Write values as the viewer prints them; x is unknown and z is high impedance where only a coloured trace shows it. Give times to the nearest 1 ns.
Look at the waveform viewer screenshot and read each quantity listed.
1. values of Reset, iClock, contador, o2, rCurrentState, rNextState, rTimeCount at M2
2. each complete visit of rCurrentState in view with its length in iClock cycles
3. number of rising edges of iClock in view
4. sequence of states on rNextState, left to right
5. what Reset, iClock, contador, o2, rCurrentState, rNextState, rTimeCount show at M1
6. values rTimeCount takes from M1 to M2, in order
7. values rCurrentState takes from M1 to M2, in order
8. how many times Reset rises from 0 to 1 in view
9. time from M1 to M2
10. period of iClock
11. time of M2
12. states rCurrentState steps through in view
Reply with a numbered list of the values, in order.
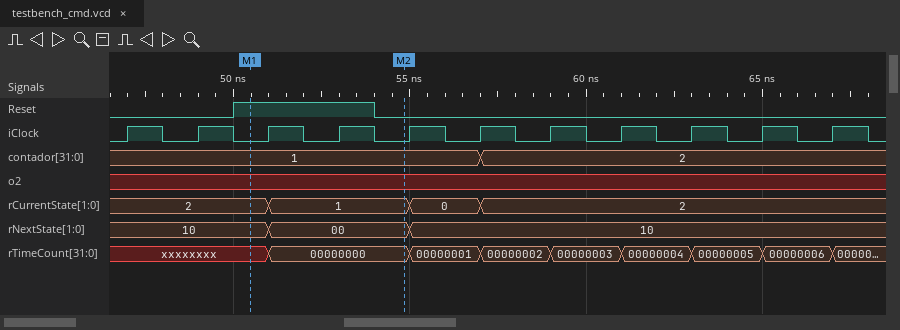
1. Reset=0, iClock=0, contador=1, o2=x, rCurrentState=1, rNextState=00, rTimeCount=00000000
2. 1: 2, 0: 1
3. 11
4. 10, 00, 10
5. Reset=1, iClock=0, contador=1, o2=x, rCurrentState=2, rNextState=10, rTimeCount=xxxxxxxx
6. xxxxxxxx, 00000000
7. 2, 1
8. 1
9. 4 ns
10. 2 ns
11. 55 ns
12. 2, 1, 0, 2
